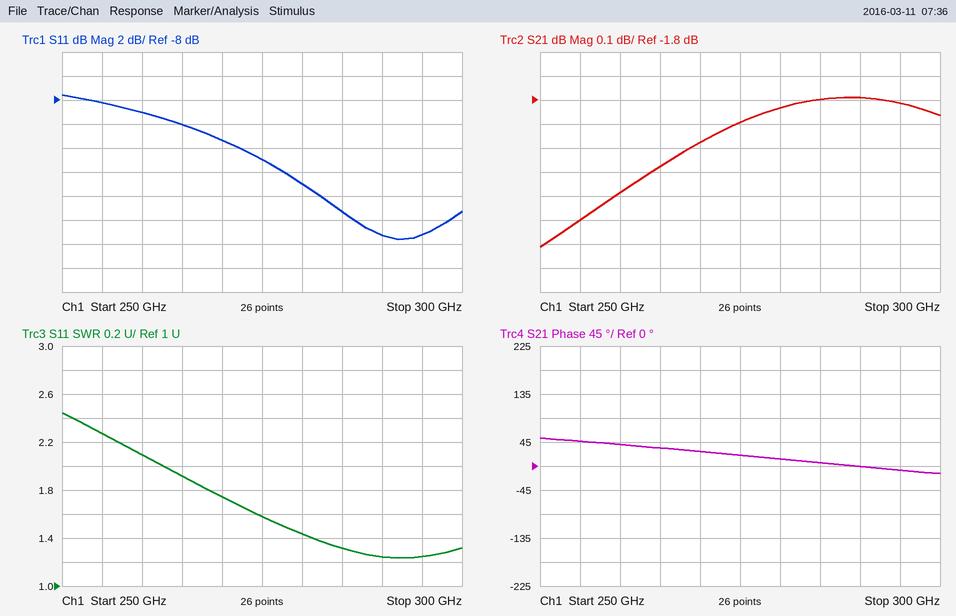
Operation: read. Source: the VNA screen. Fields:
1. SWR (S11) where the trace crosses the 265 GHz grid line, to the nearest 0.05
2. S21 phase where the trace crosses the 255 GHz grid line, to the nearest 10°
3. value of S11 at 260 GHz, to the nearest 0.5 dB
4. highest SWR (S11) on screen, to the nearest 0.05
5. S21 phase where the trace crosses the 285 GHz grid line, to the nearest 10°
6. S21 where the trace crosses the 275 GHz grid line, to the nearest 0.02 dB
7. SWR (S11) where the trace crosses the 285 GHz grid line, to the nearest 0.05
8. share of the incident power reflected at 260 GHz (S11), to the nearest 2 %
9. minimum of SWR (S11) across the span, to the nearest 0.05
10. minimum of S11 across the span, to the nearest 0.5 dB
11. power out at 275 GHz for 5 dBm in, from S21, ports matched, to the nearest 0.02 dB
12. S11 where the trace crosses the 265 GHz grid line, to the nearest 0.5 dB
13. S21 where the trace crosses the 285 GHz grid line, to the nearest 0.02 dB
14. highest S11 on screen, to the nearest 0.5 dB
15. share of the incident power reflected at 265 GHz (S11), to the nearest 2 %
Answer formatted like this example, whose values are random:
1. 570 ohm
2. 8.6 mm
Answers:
1. 1.90
2. 50°
3. -9.0 dB
4. 2.45
5. 10°
6. -1.90 dB
7. 1.30
8. 12 %
9. 1.25
10. -19.5 dB
11. 3.10 dBm
12. -10.0 dB
13. -1.80 dB
14. -7.5 dB
15. 10 %
